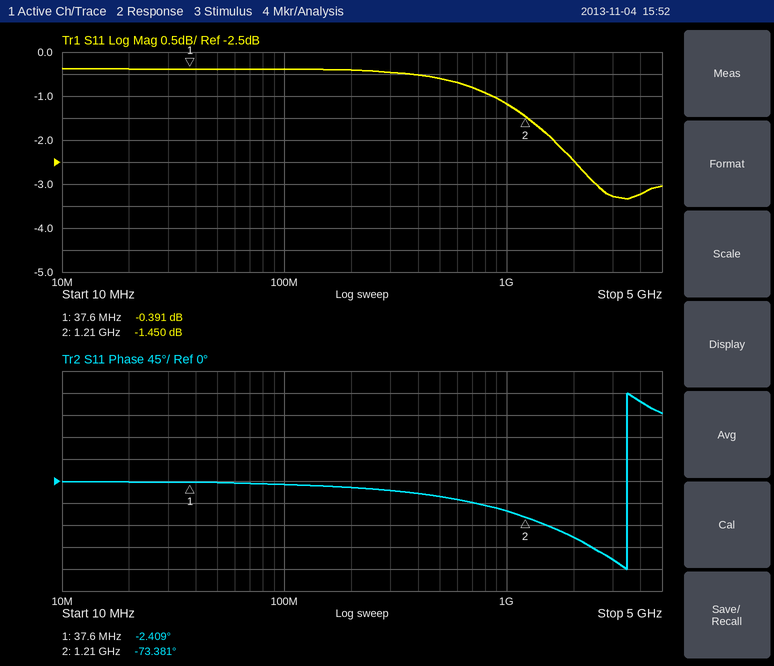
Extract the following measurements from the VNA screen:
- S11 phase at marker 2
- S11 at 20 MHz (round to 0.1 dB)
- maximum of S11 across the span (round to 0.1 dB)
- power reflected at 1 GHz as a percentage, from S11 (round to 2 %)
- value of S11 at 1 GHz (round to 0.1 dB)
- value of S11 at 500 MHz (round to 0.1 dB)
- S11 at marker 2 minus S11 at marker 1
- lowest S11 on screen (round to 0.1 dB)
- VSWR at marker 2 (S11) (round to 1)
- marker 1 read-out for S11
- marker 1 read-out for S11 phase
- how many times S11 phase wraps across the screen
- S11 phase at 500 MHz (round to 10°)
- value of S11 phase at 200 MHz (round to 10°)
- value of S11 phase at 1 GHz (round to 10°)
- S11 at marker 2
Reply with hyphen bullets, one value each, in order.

- -73.381°
- -0.4 dB
- -0.4 dB
- 76 %
- -1.2 dB
- -0.6 dB
- -1.059 dB
- -3.3 dB
- 12
- -0.391 dB
- -2.409°
- 1
- -30°
- -10°
- -60°
- -1.450 dB
